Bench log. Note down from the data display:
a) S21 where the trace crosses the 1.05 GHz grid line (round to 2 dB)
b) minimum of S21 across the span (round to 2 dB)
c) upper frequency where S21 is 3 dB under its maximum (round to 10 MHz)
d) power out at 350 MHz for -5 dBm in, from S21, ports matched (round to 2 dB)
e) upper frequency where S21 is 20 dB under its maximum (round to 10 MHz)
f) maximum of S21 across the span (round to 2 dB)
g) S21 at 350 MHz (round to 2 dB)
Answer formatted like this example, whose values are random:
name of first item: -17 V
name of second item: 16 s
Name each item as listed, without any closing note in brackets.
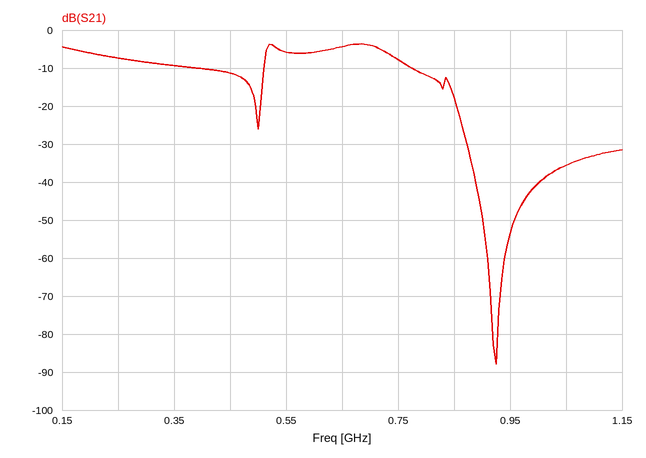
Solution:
S21 where the trace crosses the 1.05 GHz grid line: -36 dB
minimum of S21 across the span: -88 dB
upper frequency where S21 is 3 dB under its maximum: 740 MHz
power out at 350 MHz for -5 dBm in, from S21, ports matched: -14 dBm
upper frequency where S21 is 20 dB under its maximum: 860 MHz
maximum of S21 across the span: -4 dB
S21 at 350 MHz: -10 dB
